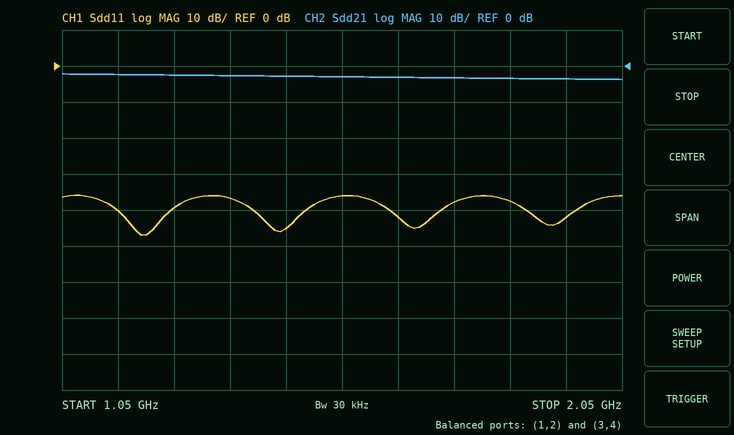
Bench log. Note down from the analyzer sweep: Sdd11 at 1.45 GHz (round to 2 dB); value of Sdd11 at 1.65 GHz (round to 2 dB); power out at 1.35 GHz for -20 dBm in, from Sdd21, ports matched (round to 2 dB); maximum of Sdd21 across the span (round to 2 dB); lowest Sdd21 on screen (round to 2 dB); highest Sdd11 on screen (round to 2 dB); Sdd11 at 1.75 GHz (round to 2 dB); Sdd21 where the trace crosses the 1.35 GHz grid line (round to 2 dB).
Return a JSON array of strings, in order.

["-46 dB", "-42 dB", "-22 dBm", "-2 dB", "-4 dB", "-36 dB", "-38 dB", "-2 dB"]
